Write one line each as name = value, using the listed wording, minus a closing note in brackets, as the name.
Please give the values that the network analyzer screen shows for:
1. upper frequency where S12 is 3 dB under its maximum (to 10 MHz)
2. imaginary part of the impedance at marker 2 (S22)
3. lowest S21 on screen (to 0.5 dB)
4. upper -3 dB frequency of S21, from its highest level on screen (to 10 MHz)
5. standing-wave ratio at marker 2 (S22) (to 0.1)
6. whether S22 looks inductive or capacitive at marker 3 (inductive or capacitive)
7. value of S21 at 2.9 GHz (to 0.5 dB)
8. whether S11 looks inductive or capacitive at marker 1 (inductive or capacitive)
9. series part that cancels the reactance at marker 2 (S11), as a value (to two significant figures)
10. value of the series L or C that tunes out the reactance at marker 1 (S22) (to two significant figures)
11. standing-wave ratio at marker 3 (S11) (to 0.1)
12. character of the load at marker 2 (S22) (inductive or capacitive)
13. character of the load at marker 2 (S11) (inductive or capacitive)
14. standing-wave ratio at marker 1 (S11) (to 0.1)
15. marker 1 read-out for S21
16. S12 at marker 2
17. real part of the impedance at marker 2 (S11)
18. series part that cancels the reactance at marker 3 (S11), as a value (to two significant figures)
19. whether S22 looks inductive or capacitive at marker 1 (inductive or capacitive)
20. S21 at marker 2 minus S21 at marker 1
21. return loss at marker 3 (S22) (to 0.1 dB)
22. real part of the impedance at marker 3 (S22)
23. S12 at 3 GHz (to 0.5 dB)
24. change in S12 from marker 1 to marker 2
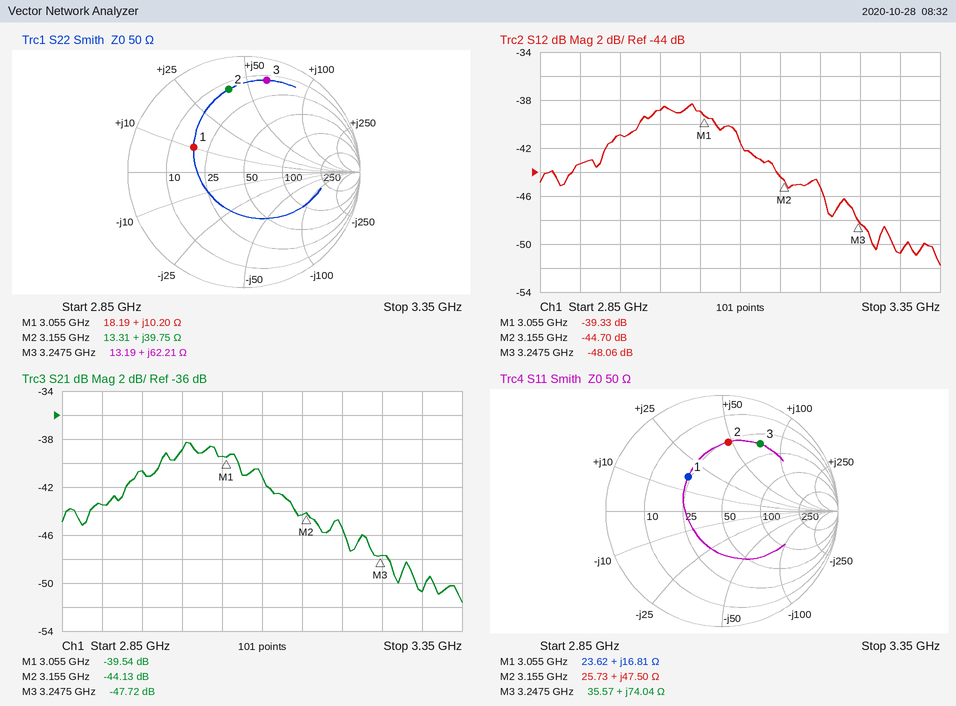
upper frequency where S12 is 3 dB under its maximum = 3.10 GHz
imaginary part of the impedance at marker 2 = +39.75 Ω
lowest S21 on screen = -51.5 dB
upper -3 dB frequency of S21, from its highest level on screen = 3.10 GHz
standing-wave ratio at marker 2 (S22) = 6.2
whether S22 looks inductive or capacitive at marker 3 = inductive
value of S21 at 2.9 GHz = -43.5 dB
whether S11 looks inductive or capacitive at marker 1 = inductive
series part that cancels the reactance at marker 2 (S11), as a value = 1.1 pF
value of the series L or C that tunes out the reactance at marker 1 (S22) = 5.1 pF
standing-wave ratio at marker 3 (S11) = 5.0
character of the load at marker 2 (S22) = inductive
character of the load at marker 2 (S11) = inductive
standing-wave ratio at marker 1 (S11) = 2.4
marker 1 read-out for S21 = -39.54 dB
S12 at marker 2 = -44.70 dB
real part of the impedance at marker 2 = 25.73 Ω
series part that cancels the reactance at marker 3 (S11), as a value = 660 fF
whether S22 looks inductive or capacitive at marker 1 = inductive
S21 at marker 2 minus S21 at marker 1 = -4.59 dB
return loss at marker 3 (S22) = 1.8 dB
real part of the impedance at marker 3 = 13.19 Ω
S12 at 3 GHz = -39.0 dB
change in S12 from marker 1 to marker 2 = -5.37 dB
